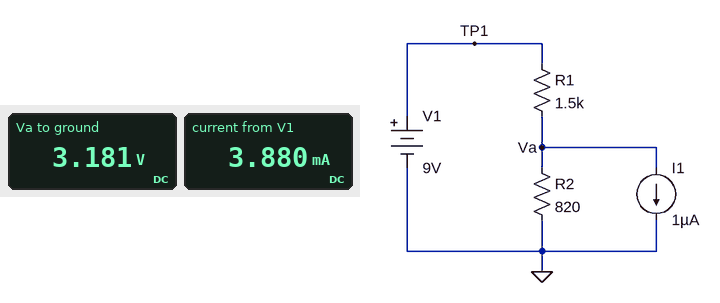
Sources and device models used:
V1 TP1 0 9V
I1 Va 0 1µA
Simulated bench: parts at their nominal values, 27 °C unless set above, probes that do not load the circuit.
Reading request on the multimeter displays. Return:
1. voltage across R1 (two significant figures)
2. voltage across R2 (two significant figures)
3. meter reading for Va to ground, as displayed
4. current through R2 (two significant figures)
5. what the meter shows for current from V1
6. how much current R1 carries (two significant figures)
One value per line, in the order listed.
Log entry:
5.8 V
3.2 V
3.181 V
3.9 mA
3.880 mA
3.9 mA
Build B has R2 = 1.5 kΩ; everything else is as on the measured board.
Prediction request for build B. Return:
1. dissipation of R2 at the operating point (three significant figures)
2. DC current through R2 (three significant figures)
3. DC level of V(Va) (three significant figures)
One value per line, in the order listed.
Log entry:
13.5 mW
3.00 mA
4.50 V
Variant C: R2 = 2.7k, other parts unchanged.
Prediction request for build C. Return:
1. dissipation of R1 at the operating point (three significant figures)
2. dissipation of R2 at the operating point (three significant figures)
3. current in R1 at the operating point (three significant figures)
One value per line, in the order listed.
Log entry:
6.89 mW
12.4 mW
2.14 mA
